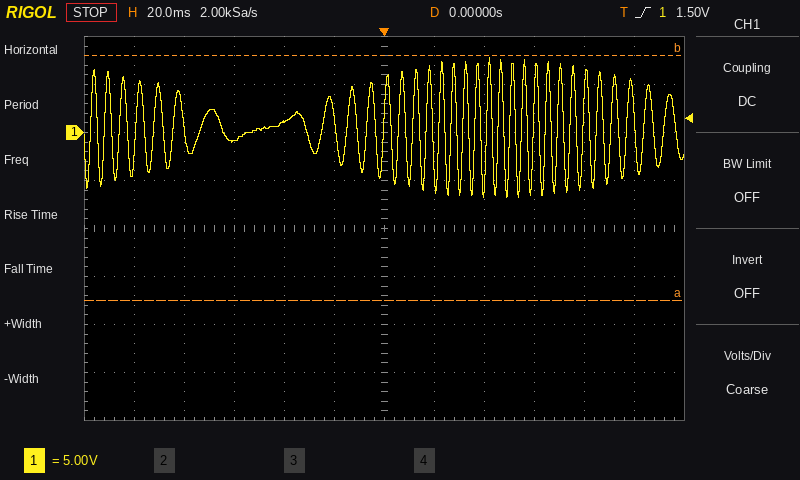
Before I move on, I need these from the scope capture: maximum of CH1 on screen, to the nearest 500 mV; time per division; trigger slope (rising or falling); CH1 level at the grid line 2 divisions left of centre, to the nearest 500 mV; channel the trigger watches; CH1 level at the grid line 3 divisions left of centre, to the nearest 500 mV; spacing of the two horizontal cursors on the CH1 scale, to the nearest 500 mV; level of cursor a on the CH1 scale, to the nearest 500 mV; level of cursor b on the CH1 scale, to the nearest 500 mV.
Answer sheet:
8.0 V
20 ms
rising
1.0 V
CH1
-1.0 V
25.5 V
-17.5 V
8.0 V
